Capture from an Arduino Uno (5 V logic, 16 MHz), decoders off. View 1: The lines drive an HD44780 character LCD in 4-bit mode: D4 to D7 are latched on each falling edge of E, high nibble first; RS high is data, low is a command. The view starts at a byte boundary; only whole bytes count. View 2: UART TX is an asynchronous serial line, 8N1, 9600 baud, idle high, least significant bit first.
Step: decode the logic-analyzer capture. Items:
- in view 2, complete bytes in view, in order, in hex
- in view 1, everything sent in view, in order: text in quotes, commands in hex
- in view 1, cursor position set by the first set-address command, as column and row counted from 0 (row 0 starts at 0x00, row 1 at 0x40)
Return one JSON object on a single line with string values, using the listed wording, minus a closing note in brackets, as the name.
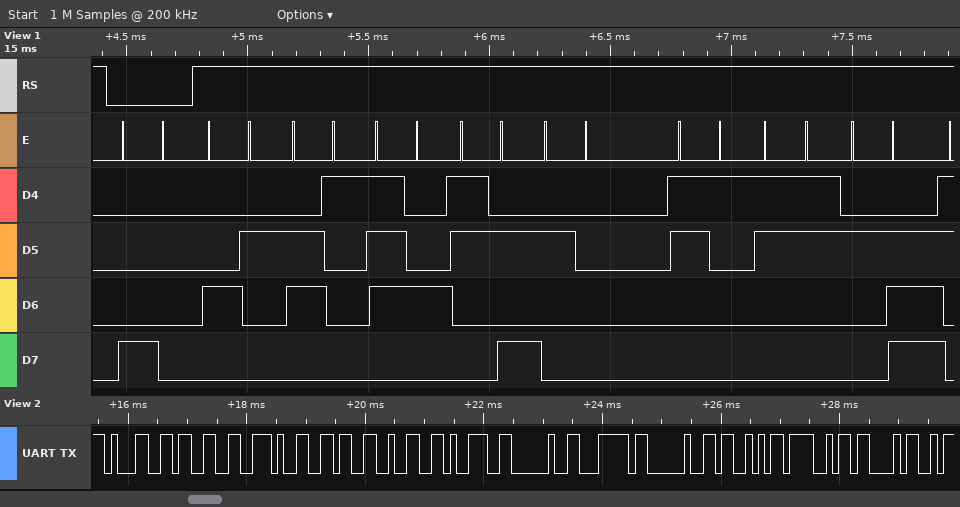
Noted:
{"in view 2, complete bytes in view, in order, in hex": "31 33 2E 36 32 39 20 7C 20 53 4F 43", "in view 1, everything sent in view, in order: text in quotes, commands in hex": "0x80 \"Bat: 13.\"", "in view 1, cursor position set by the first set-address command, as column and row counted from 0": "column 0, row 0"}
